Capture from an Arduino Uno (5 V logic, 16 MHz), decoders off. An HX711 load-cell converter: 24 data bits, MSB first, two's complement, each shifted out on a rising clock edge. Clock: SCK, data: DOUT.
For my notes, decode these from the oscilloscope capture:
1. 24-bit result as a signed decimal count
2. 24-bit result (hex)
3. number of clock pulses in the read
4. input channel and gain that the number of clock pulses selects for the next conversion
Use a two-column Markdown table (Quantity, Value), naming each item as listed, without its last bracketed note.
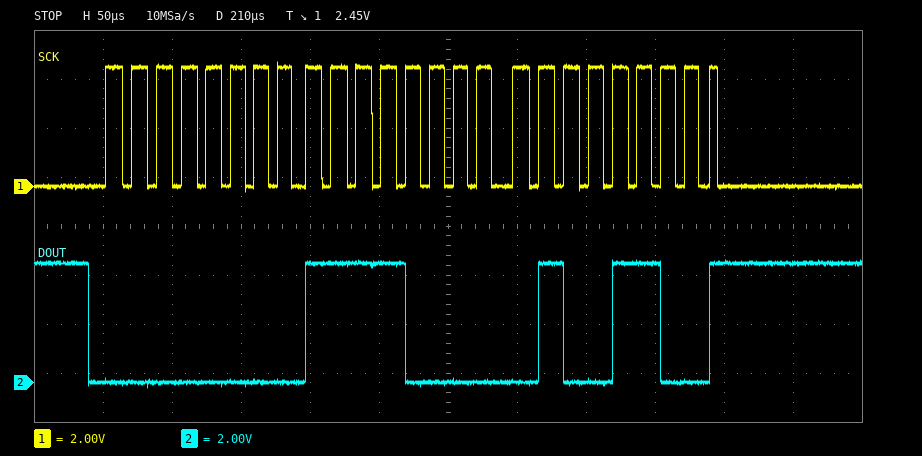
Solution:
| Quantity | Value |
|---|---|
| 24-bit result as a signed decimal count | 61516 |
| 24-bit result | 0x00F04C |
| number of clock pulses in the read | 25 |
| input channel and gain that the number of clock pulses selects for the next conversion | channel A, gain 128 |
